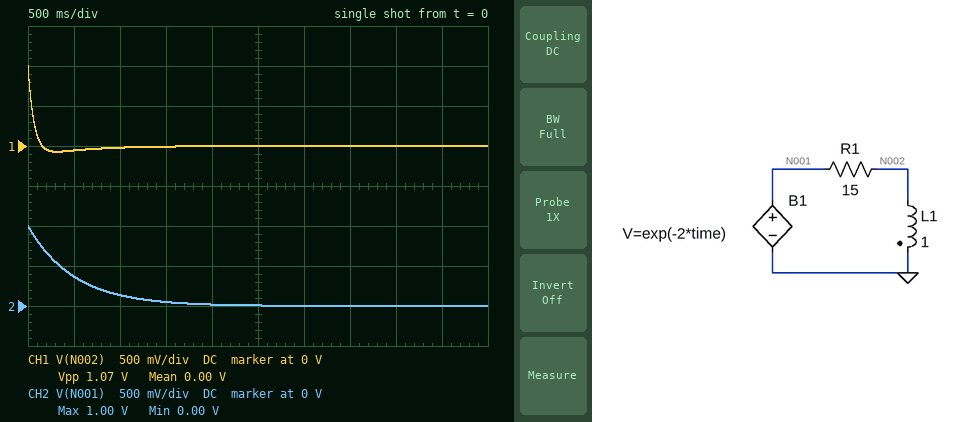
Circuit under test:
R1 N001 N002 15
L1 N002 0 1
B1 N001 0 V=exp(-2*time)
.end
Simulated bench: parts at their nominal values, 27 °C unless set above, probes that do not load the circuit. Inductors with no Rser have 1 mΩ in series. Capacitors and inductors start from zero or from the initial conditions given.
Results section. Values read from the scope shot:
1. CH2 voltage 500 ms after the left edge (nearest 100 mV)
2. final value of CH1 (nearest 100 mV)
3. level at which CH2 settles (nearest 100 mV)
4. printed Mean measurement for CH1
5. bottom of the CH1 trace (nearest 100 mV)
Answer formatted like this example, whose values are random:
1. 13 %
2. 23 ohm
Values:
1. 400 mV
2. 0 V
3. 0 V
4. 0.00 V
5. -100 mV
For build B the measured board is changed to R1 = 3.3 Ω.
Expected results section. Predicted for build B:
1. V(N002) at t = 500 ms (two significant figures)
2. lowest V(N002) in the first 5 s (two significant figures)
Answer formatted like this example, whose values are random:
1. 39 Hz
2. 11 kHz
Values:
1. -78 mV
2. -130 mV
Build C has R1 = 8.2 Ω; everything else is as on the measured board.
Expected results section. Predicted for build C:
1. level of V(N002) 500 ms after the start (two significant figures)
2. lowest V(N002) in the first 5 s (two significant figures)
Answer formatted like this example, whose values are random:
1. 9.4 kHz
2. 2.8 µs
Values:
1. -97 mV
2. -98 mV
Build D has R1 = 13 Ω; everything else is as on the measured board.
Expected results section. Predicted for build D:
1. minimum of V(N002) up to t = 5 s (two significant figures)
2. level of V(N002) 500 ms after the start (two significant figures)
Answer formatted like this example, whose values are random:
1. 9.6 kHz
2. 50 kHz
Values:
1. -78 mV
2. -65 mV
